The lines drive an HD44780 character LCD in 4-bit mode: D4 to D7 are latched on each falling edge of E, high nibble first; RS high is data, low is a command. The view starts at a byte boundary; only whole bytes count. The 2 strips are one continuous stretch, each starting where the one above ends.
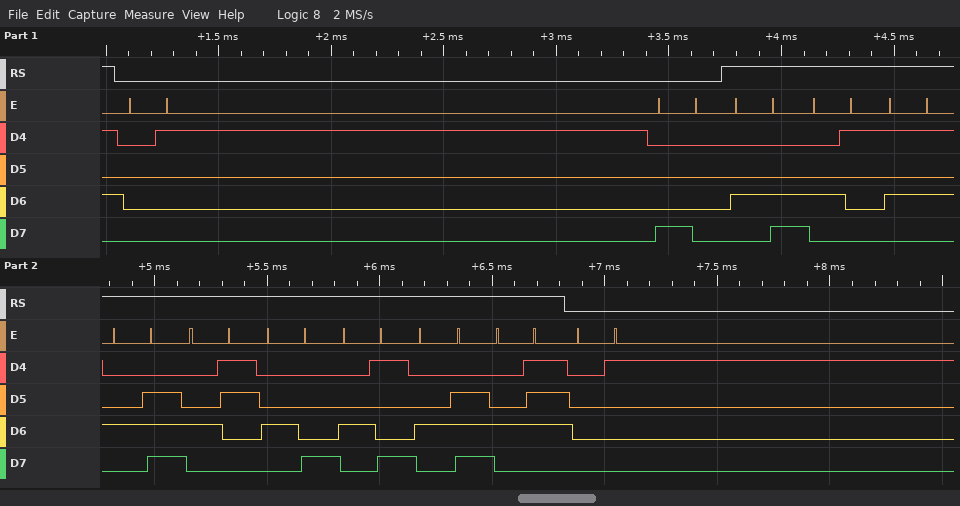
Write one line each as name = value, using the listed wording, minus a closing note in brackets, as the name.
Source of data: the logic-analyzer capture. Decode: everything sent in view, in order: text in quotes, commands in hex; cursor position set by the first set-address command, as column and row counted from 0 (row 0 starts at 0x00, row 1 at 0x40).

everything sent in view, in order: text in quotes, commands in hex = 0x01 0x80 "LAUNCHING" 0x01
cursor position set by the first set-address command, as column and row counted from 0 = column 0, row 0
